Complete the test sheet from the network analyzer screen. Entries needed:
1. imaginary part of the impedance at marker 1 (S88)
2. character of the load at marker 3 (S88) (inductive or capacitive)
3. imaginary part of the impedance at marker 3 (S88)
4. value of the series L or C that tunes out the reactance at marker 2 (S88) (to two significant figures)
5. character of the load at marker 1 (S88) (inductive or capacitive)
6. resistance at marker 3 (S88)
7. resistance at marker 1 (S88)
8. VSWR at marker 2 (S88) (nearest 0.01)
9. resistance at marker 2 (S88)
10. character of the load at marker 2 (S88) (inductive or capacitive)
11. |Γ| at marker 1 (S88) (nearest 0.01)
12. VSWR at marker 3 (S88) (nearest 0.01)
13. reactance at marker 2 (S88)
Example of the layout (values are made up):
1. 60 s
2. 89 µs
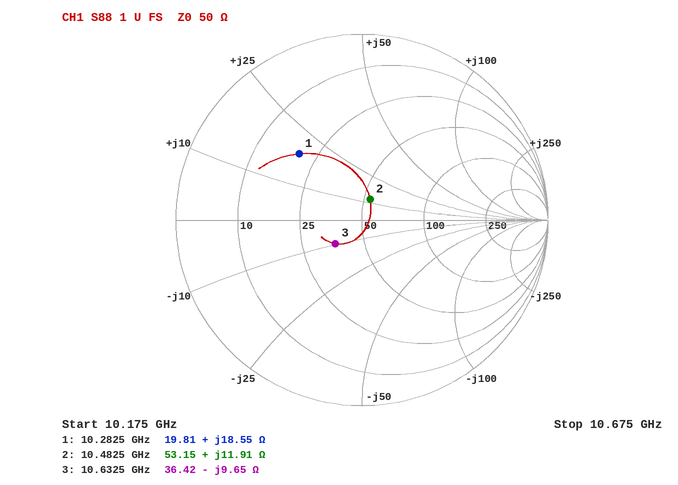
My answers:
1. +18.55 Ω
2. capacitive
3. -9.65 Ω
4. 1.3 pF
5. inductive
6. 36.42 Ω
7. 19.81 Ω
8. 1.27
9. 53.15 Ω
10. inductive
11. 0.49
12. 1.47
13. +11.91 Ω
